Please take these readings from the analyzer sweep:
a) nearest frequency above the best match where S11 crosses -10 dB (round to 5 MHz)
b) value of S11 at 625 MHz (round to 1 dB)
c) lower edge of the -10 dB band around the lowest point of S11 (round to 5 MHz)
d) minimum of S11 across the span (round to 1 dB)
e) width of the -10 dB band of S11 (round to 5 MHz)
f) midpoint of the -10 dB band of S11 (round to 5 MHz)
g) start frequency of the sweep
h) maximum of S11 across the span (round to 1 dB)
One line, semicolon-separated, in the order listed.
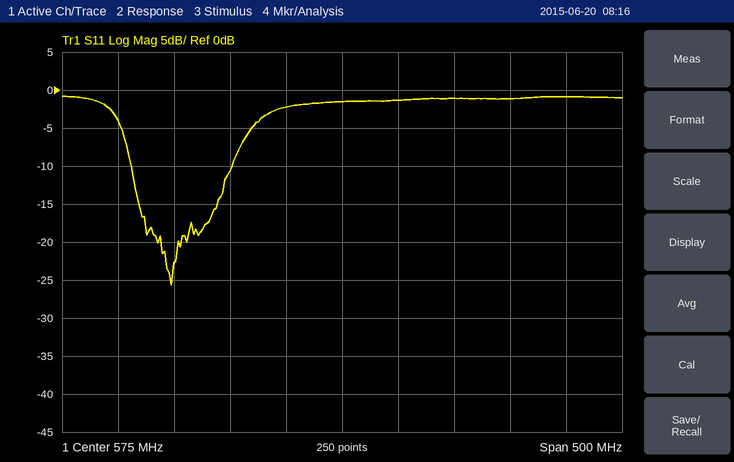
475 MHz; -1 dB; 385 MHz; -26 dB; 90 MHz; 430 MHz; 325 MHz; -1 dB
